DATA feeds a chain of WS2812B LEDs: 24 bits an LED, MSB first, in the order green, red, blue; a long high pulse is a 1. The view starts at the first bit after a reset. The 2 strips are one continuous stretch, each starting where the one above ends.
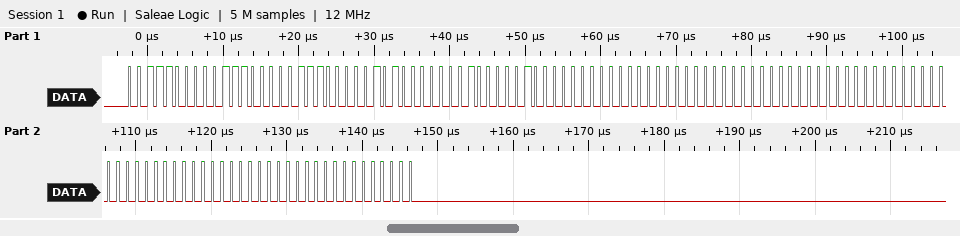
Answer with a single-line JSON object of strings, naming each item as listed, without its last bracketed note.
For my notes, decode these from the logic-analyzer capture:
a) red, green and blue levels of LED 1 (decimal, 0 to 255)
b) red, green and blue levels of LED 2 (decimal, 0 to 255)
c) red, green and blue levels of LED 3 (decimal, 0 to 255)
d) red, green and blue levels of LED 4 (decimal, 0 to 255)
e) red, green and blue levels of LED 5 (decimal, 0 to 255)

{"red, green and blue levels of LED 1": "56, 56, 56", "red, green and blue levels of LED 2": "8, 40, 32", "red, green and blue levels of LED 3": "0, 0, 0", "red, green and blue levels of LED 4": "0, 0, 0", "red, green and blue levels of LED 5": "0, 0, 0"}
